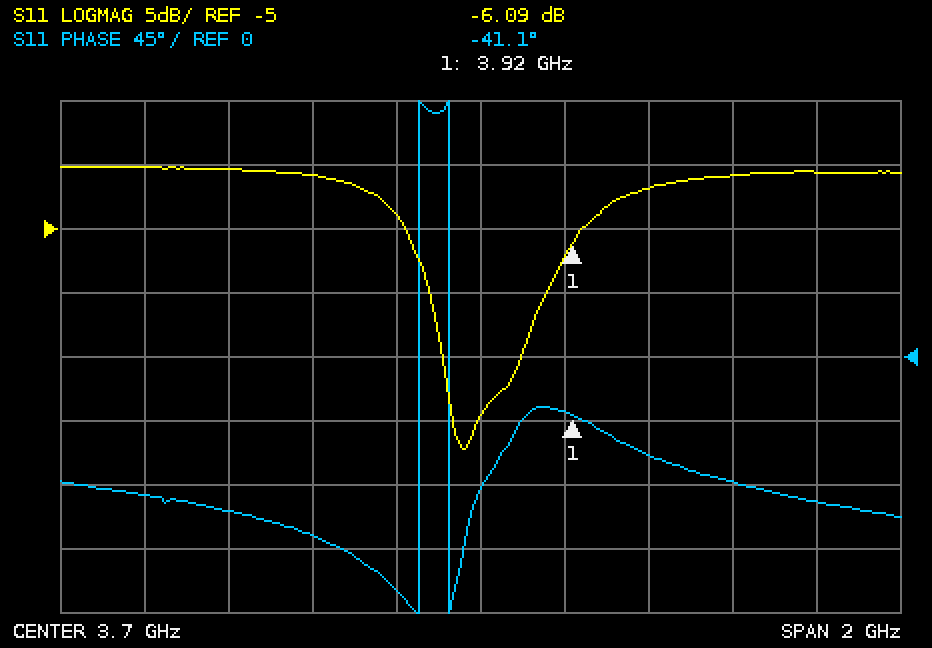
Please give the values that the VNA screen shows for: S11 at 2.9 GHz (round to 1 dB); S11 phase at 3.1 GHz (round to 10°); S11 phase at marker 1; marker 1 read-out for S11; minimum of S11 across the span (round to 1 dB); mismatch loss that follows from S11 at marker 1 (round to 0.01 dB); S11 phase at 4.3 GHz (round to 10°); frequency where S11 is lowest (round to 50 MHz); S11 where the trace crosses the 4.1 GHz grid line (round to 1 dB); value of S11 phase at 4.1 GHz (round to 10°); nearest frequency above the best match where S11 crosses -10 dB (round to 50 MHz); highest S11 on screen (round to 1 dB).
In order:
0 dB
-110°
-41.1°
-6.09 dB
-22 dB
1.23 dB
-90°
3.65 GHz
-2 dB
-70°
3.85 GHz
0 dB
